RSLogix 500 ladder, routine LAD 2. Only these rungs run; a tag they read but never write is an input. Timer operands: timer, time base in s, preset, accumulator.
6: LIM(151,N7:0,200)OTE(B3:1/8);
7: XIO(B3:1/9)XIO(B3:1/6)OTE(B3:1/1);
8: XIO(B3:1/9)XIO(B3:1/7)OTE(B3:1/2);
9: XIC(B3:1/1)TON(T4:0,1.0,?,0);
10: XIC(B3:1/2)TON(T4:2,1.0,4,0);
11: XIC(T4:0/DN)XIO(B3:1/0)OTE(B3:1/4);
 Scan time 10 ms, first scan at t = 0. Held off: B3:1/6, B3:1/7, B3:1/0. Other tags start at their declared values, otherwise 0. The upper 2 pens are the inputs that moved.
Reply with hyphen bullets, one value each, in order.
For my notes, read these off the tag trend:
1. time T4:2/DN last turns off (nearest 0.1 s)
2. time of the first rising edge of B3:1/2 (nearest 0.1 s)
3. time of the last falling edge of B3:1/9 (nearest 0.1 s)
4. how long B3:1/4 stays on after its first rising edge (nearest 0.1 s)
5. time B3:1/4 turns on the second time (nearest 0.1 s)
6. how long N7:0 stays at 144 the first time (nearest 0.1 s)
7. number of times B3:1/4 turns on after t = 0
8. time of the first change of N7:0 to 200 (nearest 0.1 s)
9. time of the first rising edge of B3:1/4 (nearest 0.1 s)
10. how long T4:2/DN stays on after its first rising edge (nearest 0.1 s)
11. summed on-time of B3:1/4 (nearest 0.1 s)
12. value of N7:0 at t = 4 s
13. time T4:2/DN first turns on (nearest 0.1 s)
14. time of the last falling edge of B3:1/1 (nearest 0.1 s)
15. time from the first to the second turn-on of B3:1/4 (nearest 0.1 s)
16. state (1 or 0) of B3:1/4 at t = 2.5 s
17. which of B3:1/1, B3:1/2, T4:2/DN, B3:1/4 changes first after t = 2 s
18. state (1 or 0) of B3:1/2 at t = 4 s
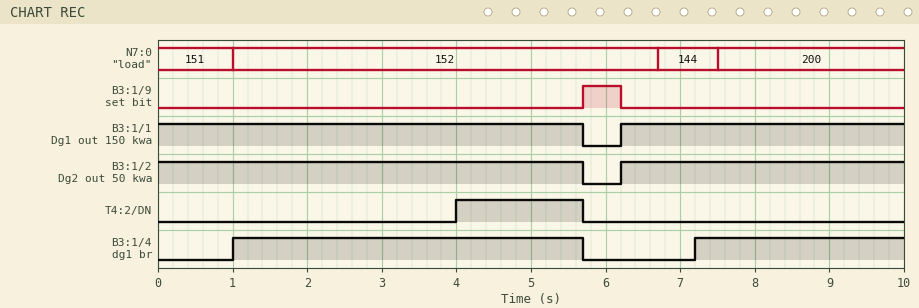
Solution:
- 5.7 s
- 6.2 s
- 6.2 s
- 4.7 s
- 7.2 s
- 0.8 s
- 2
- 7.5 s
- 1.0 s
- 1.7 s
- 7.5 s
- 152
- 4.0 s
- 5.7 s
- 6.2 s
- 1
- T4:2/DN
- 1
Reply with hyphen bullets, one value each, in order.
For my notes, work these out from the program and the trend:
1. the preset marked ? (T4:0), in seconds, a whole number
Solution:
- 1 s
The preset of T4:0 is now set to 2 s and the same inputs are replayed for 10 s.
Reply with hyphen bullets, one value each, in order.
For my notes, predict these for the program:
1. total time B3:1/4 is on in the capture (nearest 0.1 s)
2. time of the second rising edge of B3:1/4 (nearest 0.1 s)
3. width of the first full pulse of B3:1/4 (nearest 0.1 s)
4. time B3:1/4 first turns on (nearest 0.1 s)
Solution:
- 5.5 s
- 8.2 s
- 3.7 s
- 2.0 s
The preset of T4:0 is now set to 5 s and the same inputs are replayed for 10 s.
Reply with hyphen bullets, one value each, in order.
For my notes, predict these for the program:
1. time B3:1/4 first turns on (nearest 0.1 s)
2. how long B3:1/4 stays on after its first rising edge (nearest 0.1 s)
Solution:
- 5.0 s
- 0.7 s
